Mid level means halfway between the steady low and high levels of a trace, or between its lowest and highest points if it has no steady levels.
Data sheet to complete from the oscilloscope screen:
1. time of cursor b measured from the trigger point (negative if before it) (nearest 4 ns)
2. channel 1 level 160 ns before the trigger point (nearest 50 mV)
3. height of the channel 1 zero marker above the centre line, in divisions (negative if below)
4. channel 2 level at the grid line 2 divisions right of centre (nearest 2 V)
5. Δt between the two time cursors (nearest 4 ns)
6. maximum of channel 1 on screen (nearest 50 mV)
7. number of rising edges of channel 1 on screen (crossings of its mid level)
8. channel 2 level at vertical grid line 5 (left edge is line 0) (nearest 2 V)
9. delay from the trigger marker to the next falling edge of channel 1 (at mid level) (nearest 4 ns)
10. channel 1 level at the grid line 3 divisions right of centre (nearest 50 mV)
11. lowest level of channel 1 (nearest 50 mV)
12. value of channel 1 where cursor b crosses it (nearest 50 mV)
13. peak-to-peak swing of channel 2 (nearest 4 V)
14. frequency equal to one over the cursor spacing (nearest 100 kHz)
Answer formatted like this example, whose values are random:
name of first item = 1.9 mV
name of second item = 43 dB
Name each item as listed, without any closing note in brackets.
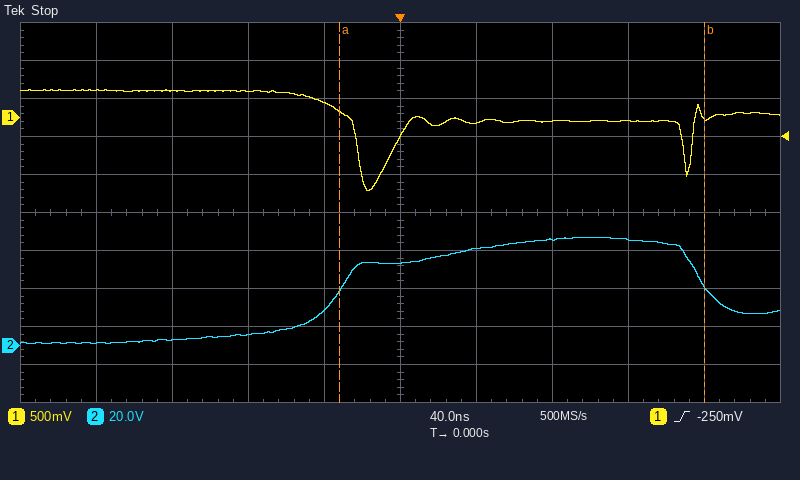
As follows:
time of cursor b measured from the trigger point (negative if before it) = +160 ns
channel 1 level 160 ns before the trigger point = 350 mV
height of the channel 1 zero marker above the centre line, in divisions = +2.5 div
channel 2 level at the grid line 2 divisions right of centre = 56 V
Δt between the two time cursors = 192 ns
maximum of channel 1 on screen = 350 mV
number of rising edges of channel 1 on screen = 2
channel 2 level at vertical grid line 5 (left edge is line 0) = 44 V
delay from the trigger marker to the next falling edge of channel 1 (at mid level) = 148 ns
channel 1 level at the grid line 3 divisions right of centre = -50 mV
lowest level of channel 1 = -950 mV
value of channel 1 where cursor b crosses it = 0 mV
peak-to-peak swing of channel 2 = 56 V
frequency equal to one over the cursor spacing = 5.2 MHz
